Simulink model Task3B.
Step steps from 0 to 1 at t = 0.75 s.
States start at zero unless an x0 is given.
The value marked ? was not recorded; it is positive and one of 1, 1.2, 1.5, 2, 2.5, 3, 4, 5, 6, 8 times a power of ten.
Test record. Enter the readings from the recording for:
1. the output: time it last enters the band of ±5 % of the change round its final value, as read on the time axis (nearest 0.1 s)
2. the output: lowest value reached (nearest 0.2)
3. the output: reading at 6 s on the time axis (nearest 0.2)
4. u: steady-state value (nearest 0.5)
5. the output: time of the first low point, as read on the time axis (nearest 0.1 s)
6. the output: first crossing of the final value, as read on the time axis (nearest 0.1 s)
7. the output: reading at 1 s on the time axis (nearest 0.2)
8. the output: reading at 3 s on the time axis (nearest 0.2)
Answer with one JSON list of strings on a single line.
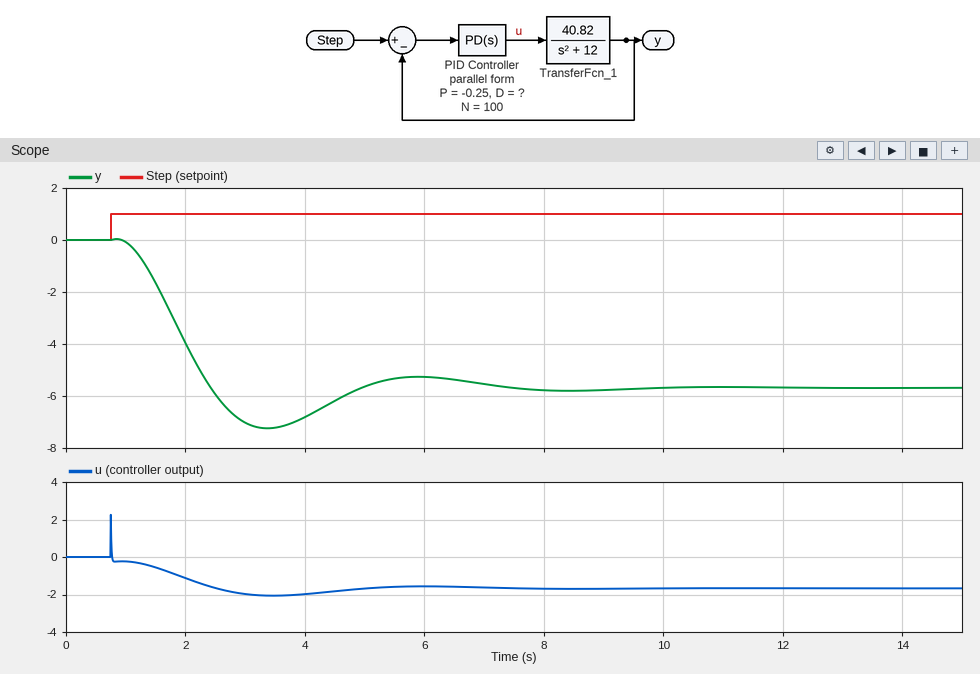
["6.6 s", "-7.2", "-5.2", "-1.5", "3.4 s", "2.4 s", "0.0", "-7.0"]
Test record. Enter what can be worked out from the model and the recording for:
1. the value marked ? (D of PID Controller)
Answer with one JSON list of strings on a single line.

["0.025"]
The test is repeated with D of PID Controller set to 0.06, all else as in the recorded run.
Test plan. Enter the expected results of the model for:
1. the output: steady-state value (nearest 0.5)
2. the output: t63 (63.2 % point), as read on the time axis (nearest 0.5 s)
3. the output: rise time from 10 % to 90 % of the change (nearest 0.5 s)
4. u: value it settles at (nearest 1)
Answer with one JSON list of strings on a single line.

["-5.5", "2.5 s", "2.0 s", "-2"]
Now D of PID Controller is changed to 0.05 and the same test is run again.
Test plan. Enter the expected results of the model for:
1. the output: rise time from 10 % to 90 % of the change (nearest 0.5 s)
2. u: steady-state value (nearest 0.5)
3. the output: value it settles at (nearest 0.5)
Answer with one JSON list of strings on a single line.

["1.5 s", "-1.5", "-5.5"]
